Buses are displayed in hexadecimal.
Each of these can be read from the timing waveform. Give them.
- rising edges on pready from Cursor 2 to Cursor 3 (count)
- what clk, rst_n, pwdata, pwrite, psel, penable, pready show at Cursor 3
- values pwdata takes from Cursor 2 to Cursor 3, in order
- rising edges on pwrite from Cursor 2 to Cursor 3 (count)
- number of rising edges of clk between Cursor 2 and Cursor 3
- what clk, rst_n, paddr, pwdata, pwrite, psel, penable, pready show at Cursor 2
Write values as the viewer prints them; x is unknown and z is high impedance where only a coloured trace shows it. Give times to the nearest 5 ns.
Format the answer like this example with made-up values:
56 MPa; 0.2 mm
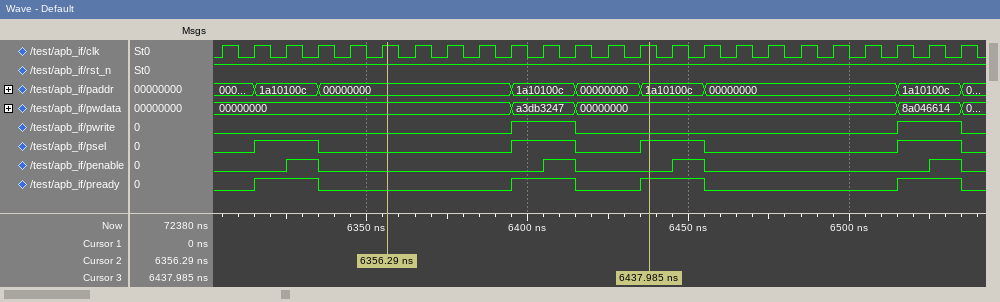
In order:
2; clk=1, rst_n=1, pwdata=00000000, pwrite=0, psel=1, penable=0, pready=1; 00000000, a3db3247, 00000000; 1; 8; clk=1, rst_n=1, paddr=00000000, pwdata=00000000, pwrite=0, psel=0, penable=0, pready=0
